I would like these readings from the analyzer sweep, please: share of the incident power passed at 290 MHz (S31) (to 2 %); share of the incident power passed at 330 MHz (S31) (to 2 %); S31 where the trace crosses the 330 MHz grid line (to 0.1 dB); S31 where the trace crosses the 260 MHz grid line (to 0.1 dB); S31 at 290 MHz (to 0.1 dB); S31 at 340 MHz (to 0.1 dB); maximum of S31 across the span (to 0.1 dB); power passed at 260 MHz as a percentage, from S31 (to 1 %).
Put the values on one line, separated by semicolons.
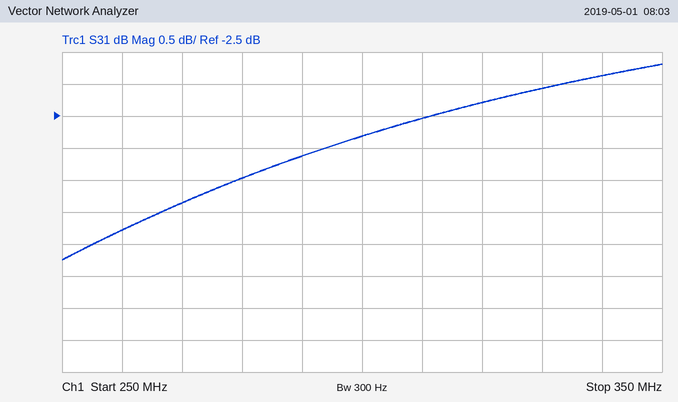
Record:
48 %; 62 %; -2.1 dB; -4.3 dB; -3.1 dB; -1.9 dB; -1.7 dB; 37 %
